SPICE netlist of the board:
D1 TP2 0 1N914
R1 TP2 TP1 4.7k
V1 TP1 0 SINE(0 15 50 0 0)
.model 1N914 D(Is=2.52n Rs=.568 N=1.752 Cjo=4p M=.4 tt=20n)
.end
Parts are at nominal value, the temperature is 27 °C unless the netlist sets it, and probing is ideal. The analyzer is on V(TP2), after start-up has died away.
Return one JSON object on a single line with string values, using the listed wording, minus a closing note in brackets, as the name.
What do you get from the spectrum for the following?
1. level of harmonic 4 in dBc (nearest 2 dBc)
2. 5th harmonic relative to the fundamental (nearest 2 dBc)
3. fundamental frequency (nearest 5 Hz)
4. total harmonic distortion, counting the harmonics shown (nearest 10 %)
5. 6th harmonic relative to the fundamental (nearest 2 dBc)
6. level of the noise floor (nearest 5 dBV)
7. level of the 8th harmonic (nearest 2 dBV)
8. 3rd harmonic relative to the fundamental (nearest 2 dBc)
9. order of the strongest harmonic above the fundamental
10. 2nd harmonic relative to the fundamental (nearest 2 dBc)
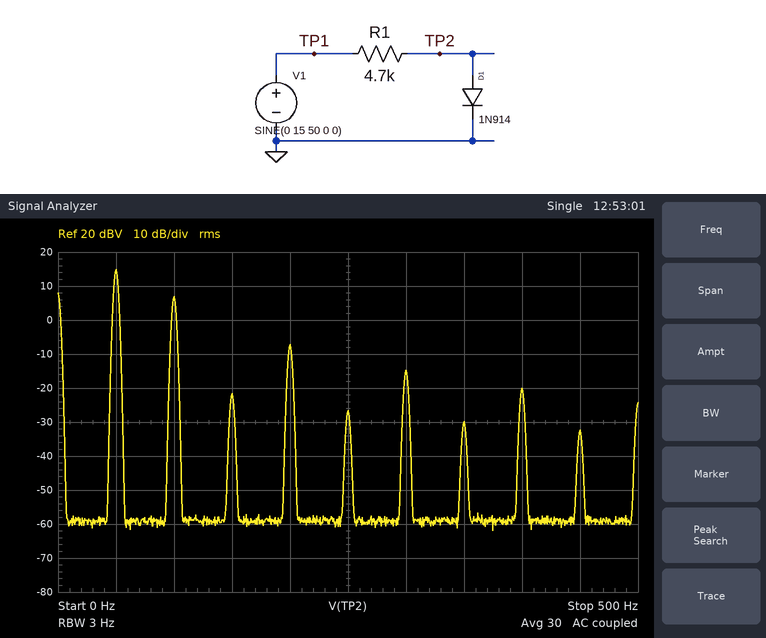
{"level of harmonic 4 in dBc": "-22 dBc", "5th harmonic relative to the fundamental": "-42 dBc", "fundamental frequency": "50 Hz", "total harmonic distortion, counting the harmonics shown": "40 %", "6th harmonic relative to the fundamental": "-30 dBc", "level of the noise floor": "-60 dBV", "level of the 8th harmonic": "-20 dBV", "3rd harmonic relative to the fundamental": "-36 dBc", "order of the strongest harmonic above the fundamental": "2", "2nd harmonic relative to the fundamental": "-8 dBc"}
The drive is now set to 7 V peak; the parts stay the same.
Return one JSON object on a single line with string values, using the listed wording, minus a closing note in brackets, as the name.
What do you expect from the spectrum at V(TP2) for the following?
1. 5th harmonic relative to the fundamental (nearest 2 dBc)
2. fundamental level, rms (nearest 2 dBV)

{"5th harmonic relative to the fundamental": "-36 dBc", "fundamental level, rms": "8 dBV"}
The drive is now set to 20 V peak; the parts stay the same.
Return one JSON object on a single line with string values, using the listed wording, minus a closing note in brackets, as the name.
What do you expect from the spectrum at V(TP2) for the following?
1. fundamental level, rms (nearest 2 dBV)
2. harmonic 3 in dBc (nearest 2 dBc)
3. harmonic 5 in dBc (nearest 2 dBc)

{"fundamental level, rms": "18 dBV", "harmonic 3 in dBc": "-38 dBc", "harmonic 5 in dBc": "-44 dBc"}
